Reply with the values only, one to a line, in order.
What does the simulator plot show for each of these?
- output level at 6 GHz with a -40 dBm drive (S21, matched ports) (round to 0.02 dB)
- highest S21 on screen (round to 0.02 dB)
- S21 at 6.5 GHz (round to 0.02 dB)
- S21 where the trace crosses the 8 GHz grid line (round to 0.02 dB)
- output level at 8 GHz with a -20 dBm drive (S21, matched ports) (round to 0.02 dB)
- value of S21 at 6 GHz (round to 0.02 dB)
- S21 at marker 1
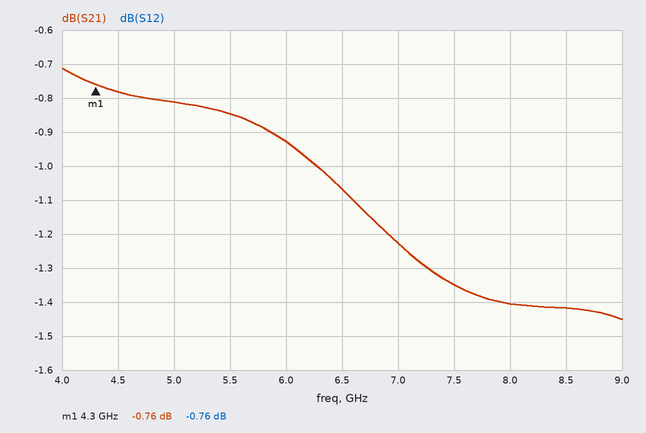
-40.92 dBm
-0.72 dB
-1.06 dB
-1.40 dB
-21.40 dBm
-0.92 dB
-0.76 dB
